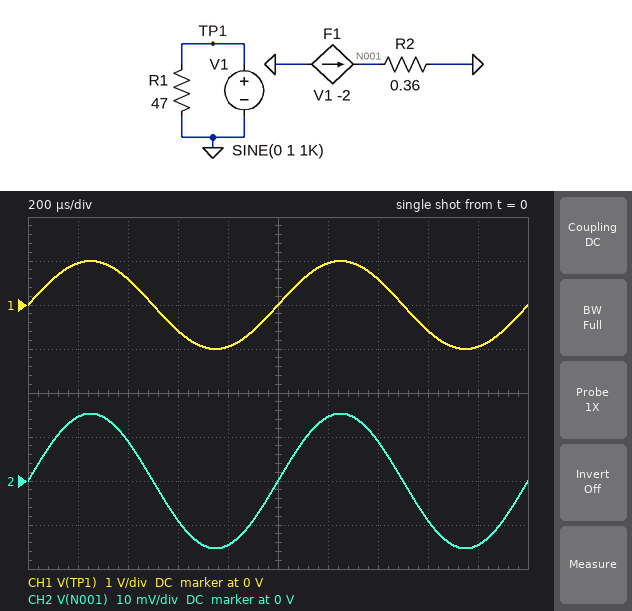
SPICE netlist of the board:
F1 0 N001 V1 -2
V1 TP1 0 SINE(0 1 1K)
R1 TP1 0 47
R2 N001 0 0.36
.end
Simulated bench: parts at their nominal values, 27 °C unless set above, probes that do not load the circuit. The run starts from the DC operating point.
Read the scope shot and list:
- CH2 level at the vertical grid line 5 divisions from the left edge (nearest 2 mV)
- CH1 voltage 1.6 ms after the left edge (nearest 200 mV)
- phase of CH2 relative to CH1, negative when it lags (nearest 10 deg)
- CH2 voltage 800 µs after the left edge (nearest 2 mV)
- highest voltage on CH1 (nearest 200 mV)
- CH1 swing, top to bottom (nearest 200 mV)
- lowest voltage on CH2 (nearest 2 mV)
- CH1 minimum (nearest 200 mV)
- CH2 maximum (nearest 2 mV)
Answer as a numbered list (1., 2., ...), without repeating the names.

1. 0 V
2. -600 mV
3. 0 deg
4. -14 mV
5. 1.0 V
6. 2.0 V
7. -16 mV
8. -1.0 V
9. 16 mV
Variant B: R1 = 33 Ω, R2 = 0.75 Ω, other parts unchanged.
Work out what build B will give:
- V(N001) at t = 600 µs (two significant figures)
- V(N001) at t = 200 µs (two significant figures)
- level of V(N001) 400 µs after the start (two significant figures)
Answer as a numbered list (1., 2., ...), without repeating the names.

1. -27 mV
2. 43 mV
3. 27 mV
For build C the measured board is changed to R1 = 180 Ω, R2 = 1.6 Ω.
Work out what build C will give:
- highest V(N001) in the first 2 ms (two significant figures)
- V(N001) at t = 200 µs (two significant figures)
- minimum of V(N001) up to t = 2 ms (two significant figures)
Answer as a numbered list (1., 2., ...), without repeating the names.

1. 18 mV
2. 17 mV
3. -18 mV
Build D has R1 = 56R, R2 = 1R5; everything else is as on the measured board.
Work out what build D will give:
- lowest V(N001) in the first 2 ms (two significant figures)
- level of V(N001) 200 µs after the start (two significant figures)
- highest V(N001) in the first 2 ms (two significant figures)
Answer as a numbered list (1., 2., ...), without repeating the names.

1. -54 mV
2. 51 mV
3. 54 mV
